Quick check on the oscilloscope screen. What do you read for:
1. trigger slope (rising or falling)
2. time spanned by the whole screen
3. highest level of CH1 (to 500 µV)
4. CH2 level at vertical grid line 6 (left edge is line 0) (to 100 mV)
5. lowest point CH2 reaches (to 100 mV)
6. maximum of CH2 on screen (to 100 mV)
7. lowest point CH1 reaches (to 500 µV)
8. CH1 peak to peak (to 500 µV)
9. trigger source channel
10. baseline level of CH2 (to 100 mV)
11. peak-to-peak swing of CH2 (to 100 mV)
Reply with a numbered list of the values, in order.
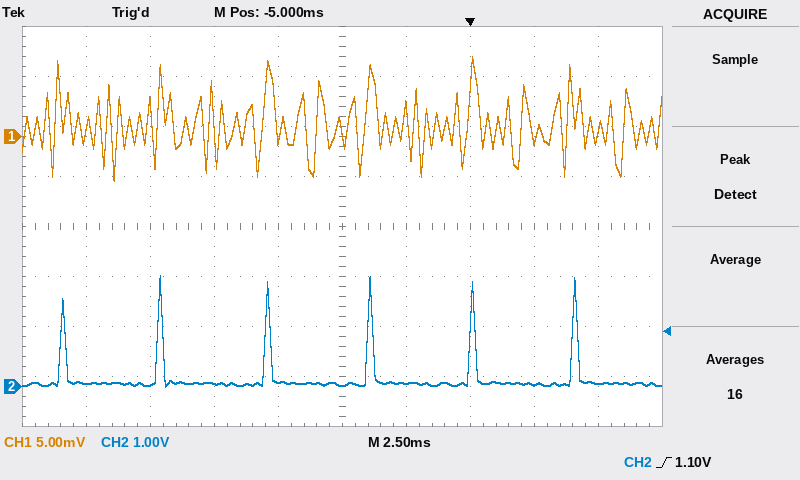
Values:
1. rising
2. 25 ms
3. 8.0 mV
4. 100 mV
5. 0.0 V
6. 2.2 V
7. -4.5 mV
8. 12.5 mV
9. CH2
10. 100 mV
11. 2.2 V
